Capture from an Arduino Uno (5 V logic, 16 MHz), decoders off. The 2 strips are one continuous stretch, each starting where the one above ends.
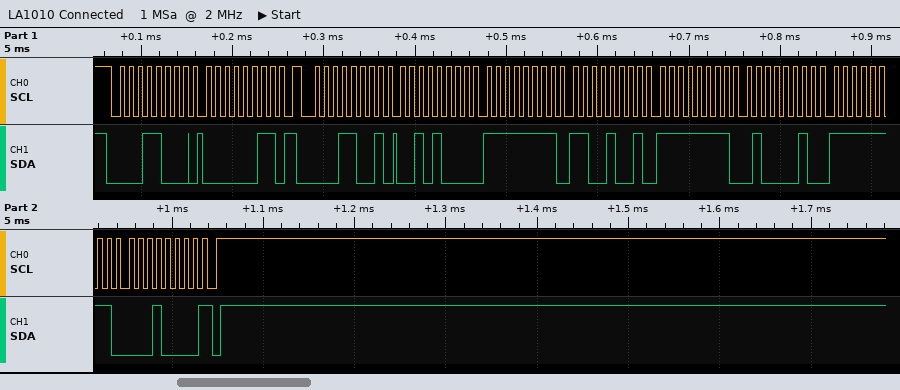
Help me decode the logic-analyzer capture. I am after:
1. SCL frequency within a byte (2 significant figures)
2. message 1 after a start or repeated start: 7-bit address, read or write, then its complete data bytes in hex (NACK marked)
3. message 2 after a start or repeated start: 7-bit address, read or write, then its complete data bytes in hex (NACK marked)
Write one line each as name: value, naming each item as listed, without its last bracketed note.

SCL frequency within a byte: 100 kHz
message 1 after a start or repeated start: 7-bit address, read or write, then its complete data bytes in hex: 0x0C write: 03
message 2 after a start or repeated start: 7-bit address, read or write, then its complete data bytes in hex: 0x0C read: 28 FF C9 FF 42 FF 10 NACK
